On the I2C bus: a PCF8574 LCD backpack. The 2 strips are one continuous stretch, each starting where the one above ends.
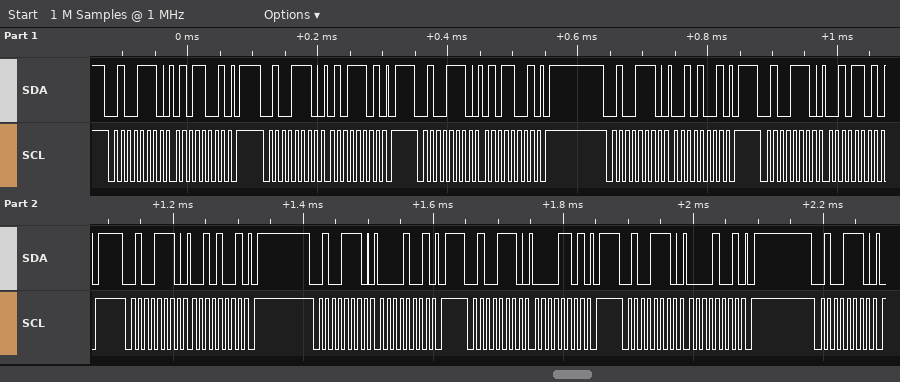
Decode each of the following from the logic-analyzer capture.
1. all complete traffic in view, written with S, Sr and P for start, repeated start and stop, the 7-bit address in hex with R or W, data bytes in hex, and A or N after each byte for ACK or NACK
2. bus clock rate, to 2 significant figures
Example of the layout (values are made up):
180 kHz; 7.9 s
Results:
S 27W A 59 A P S 27W A 5D A P S 27W A 59 A P S 27W A 29 A P S 27W A 2D A P S 27W A 29 A P S 27W A 09 A P S 27W A 0D A P S 27W A 09 A P S 27W A; 100 kHz
